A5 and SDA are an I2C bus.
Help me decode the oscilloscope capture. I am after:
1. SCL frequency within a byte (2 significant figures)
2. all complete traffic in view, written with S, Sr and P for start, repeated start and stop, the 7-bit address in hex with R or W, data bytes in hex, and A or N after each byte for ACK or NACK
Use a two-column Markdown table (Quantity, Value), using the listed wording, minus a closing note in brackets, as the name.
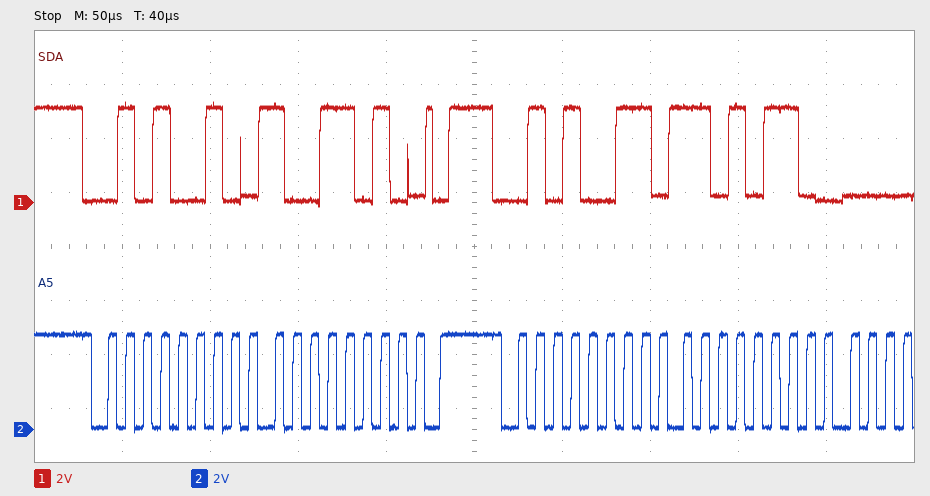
| Quantity | Value |
|---|---|
| SCL frequency within a byte | 100 kHz |
| all complete traffic in view, written with S, Sr and P for start, repeated start and stop, the 7-bit address in hex with R or W, data bytes in hex, and A or N after each byte for ACK or NACK | S 29W A 9A A P S 29R A D6 A |
